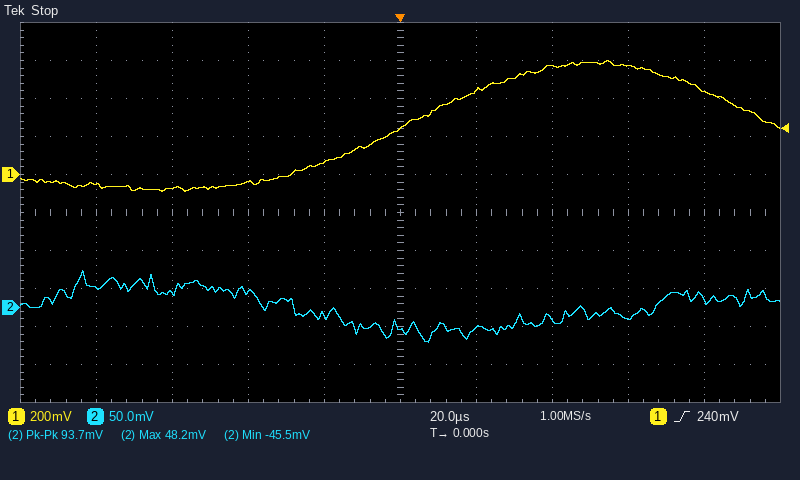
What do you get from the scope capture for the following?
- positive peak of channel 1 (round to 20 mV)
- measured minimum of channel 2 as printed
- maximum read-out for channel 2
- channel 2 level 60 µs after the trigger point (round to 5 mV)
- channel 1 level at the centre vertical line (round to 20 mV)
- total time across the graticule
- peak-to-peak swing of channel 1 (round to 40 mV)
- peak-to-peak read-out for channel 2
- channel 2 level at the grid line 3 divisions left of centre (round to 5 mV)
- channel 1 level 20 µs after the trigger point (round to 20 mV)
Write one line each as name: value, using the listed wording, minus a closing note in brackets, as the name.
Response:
positive peak of channel 1: 600 mV
measured minimum of channel 2 as printed: -45.5 mV
maximum read-out for channel 2: 48.2 mV
channel 2 level 60 µs after the trigger point: -15 mV
channel 1 level at the centre vertical line: 240 mV
total time across the graticule: 200 µs
peak-to-peak swing of channel 1: 680 mV
peak-to-peak read-out for channel 2: 93.7 mV
channel 2 level at the grid line 3 divisions left of centre: 20 mV
channel 1 level 20 µs after the trigger point: 440 mV
